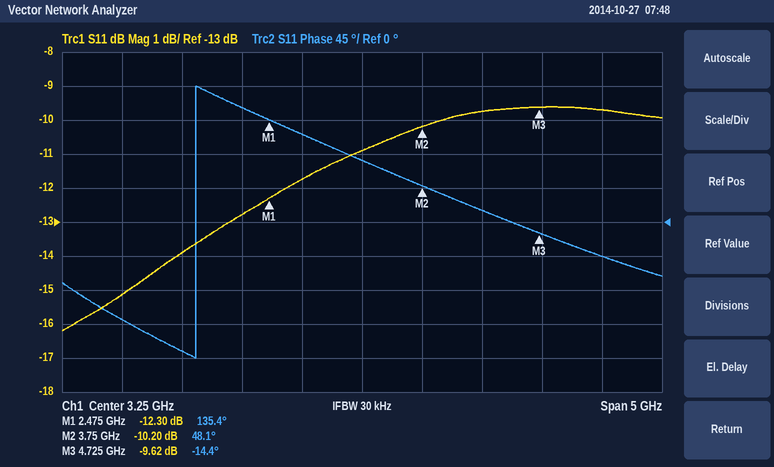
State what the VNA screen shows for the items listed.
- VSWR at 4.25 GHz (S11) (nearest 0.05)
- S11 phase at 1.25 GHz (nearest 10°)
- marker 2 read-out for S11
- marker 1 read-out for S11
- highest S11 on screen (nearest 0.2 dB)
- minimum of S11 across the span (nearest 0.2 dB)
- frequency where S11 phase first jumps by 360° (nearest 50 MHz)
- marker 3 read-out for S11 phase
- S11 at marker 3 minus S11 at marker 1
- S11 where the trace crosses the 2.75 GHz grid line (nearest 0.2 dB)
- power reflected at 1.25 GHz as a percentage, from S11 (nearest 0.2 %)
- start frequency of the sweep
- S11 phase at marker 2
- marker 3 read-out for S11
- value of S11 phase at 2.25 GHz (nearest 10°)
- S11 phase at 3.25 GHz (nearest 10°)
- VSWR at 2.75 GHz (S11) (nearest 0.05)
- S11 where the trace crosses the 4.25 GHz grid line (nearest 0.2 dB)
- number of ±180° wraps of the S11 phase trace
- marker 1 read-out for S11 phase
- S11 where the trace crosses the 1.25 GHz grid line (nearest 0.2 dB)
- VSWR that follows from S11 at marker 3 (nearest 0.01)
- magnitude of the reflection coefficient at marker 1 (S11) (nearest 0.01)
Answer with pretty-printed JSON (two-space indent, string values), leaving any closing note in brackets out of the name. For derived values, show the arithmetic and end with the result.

{
  "VSWR at 4.25 GHz (S11)": "|Γ| = 10^(-9.8/20) = 0.3236; VSWR = (1 + 0.3236)/(1 − 0.3236) ≈ 1.96, so 1.95 to the nearest 0.05",
  "S11 phase at 1.25 GHz": "-130°",
  "marker 2 read-out for S11": "-10.20 dB",
  "marker 1 read-out for S11": "-12.30 dB",
  "highest S11 on screen": "-9.6 dB",
  "minimum of S11 across the span": "-16.2 dB",
  "frequency where S11 phase first jumps by 360°": "1.85 GHz",
  "marker 3 read-out for S11 phase": "-14.4°",
  "S11 at marker 3 minus S11 at marker 1": "-9.62 − (-12.3) = 2.68 dB",
  "S11 where the trace crosses the 2.75 GHz grid line": "-11.8 dB",
  "power reflected at 1.25 GHz as a percentage, from S11": "10^(-15.2/10) ≈ 3.0 %",
  "start frequency of the sweep": "750 MHz",
  "S11 phase at marker 2": "48.1°",
  "marker 3 read-out for S11": "-9.62 dB",
  "value of S11 phase at 2.25 GHz": "150°",
  "S11 phase at 3.25 GHz": "80°",
  "VSWR at 2.75 GHz (S11)": "|Γ| = 10^(-11.8/20) = 0.2570; VSWR = (1 + 0.2570)/(1 − 0.2570) ≈ 1.69, so 1.70 to the nearest 0.05",
  "S11 where the trace crosses the 4.25 GHz grid line": "-9.8 dB",
  "number of ±180° wraps of the S11 phase trace": "1",
  "marker 1 read-out for S11 phase": "135.4°",
  "S11 where the trace crosses the 1.25 GHz grid line": "-15.2 dB",
  "VSWR that follows from S11 at marker 3": "(1 + 0.3304)/(1 − 0.3304) ≈ 1.99",
  "magnitude of the reflection coefficient at marker 1 (S11)": "10^(-12.3/20) ≈ 0.24"
}
